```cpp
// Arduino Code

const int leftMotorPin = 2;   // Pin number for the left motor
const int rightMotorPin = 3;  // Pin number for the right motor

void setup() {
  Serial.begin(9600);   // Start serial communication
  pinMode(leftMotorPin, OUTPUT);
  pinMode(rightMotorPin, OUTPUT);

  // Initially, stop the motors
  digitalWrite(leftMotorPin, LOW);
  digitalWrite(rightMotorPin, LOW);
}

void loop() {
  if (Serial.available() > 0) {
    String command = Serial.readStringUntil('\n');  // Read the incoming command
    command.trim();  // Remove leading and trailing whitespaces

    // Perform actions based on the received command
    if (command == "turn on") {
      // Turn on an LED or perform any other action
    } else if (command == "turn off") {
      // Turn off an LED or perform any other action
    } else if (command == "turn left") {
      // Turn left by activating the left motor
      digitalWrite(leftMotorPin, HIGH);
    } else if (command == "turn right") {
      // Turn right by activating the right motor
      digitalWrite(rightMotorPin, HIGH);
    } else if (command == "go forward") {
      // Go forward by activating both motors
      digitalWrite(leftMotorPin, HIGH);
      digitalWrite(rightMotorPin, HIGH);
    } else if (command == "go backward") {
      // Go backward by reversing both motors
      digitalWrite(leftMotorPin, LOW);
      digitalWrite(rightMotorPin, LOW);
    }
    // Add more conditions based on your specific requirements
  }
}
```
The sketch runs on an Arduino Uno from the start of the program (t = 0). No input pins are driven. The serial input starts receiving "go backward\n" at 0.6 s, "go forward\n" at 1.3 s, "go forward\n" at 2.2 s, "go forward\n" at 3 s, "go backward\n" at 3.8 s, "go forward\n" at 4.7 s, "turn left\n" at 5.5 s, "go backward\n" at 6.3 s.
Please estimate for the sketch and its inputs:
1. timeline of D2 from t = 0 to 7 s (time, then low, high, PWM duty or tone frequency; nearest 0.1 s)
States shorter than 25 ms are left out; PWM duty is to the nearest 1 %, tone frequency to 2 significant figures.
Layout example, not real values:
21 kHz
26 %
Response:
0 s low; 1.3 s high; 3.8 s low; 4.7 s high; 6.3 s low
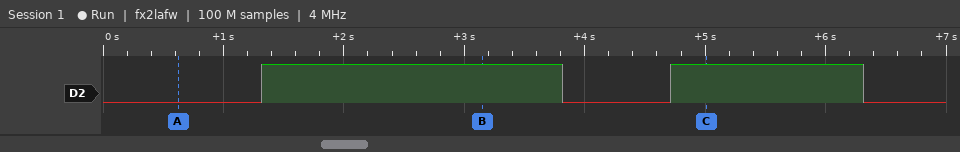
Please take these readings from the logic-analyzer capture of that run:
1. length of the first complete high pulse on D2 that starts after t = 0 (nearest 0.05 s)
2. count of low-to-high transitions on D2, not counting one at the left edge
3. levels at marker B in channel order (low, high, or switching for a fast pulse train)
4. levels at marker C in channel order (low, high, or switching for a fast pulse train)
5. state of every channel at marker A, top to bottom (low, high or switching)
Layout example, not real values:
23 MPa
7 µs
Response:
2.50 s
2
D2 high
D2 high
D2 low
